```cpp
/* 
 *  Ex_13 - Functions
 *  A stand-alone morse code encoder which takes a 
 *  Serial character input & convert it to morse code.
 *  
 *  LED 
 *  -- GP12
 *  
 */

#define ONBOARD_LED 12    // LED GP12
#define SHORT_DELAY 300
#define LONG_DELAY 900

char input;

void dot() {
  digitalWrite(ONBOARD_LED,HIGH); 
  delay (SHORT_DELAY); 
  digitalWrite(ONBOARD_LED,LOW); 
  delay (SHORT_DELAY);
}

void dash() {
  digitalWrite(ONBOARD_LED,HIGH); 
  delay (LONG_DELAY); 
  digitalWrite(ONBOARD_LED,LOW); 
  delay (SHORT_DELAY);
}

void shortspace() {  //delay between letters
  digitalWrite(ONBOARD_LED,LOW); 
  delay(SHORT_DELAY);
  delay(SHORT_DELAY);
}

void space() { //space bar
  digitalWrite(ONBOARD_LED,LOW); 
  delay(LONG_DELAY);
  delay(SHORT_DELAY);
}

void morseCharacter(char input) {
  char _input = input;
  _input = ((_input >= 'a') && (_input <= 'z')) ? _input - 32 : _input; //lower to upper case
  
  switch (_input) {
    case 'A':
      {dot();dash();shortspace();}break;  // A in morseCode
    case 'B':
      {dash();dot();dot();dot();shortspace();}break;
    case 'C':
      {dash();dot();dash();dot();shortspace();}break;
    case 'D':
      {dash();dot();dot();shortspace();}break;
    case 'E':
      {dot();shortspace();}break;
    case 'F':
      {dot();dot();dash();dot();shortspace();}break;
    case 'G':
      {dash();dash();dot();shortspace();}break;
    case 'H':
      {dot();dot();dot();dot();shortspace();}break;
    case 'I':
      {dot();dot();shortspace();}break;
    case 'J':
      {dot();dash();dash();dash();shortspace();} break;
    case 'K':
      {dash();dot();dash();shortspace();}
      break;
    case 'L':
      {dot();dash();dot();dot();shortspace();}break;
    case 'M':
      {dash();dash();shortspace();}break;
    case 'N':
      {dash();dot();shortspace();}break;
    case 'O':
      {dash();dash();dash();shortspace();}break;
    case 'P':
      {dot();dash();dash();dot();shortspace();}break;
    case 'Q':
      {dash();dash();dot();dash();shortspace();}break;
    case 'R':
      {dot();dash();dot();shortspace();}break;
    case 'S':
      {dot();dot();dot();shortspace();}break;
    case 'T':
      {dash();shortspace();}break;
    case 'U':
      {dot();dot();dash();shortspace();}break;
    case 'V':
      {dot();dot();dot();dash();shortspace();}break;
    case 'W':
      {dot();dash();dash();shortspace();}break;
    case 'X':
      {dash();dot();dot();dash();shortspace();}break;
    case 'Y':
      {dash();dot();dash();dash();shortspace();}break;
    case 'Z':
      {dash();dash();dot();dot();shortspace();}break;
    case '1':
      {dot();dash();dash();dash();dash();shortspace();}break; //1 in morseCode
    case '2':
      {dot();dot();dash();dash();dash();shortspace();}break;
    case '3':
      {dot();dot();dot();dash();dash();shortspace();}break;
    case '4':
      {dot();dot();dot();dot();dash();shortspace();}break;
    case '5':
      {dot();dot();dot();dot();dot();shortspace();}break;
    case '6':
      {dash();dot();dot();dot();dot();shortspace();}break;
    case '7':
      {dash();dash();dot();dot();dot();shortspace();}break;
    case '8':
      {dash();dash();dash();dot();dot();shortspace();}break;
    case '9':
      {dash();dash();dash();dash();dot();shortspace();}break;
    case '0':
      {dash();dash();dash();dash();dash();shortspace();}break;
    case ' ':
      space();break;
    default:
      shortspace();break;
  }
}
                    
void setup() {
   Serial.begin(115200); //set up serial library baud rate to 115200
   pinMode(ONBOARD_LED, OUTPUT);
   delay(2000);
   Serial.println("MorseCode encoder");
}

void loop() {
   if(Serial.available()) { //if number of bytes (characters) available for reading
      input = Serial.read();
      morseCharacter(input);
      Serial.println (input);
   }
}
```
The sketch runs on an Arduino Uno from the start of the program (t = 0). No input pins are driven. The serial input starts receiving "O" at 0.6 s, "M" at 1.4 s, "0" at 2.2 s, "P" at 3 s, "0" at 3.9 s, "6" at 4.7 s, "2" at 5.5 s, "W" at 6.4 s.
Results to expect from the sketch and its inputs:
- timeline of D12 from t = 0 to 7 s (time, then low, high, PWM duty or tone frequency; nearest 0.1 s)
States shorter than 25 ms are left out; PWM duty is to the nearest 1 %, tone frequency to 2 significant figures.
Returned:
0 s low; 2 s high; 2.9 s low; 3.2 s high; 4.1 s low; 4.4 s high; 5.3 s low; 6.2 s high
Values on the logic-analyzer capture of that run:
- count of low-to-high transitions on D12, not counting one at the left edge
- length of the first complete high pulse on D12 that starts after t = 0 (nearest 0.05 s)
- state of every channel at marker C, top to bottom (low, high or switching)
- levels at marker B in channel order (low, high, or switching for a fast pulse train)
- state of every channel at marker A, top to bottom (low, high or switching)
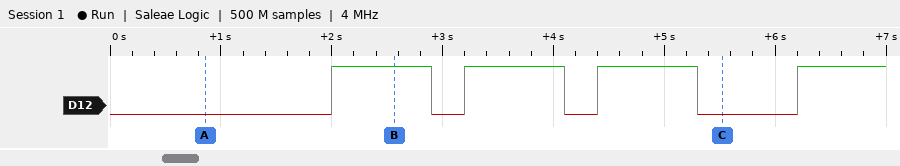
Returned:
4
0.90 s
D12 low
D12 high
D12 low
